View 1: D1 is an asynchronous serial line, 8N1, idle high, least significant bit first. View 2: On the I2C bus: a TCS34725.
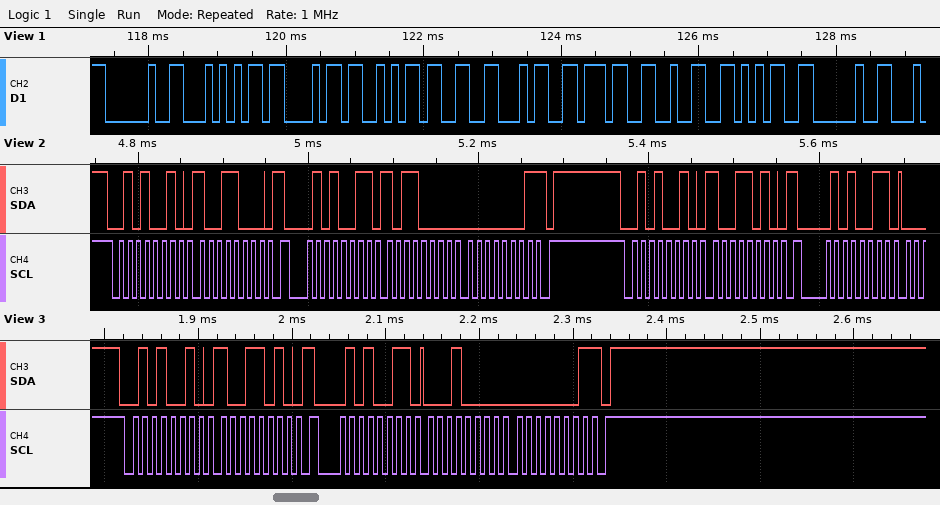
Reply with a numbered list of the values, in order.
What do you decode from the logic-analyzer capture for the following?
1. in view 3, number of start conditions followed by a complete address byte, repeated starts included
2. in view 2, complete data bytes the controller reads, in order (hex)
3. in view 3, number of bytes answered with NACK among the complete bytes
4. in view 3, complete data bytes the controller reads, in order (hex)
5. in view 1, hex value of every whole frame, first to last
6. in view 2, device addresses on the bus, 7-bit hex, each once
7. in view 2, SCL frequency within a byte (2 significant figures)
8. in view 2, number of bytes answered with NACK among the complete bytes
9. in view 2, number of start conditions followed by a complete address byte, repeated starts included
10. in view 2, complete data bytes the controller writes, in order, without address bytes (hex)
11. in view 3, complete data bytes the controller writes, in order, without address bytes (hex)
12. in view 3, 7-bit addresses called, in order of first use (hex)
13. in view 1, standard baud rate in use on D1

1. 2
2. B0 01
3. 1
4. 10 01
5. 0x20 0x54 0x43 0x53 0x33 0x34 0x37 0x32 0x35 0x20
6. 0x29
7. 100 kHz
8. 1
9. 4
10. 98 9A
11. 9A
12. 0x29
13. 9600 baud
